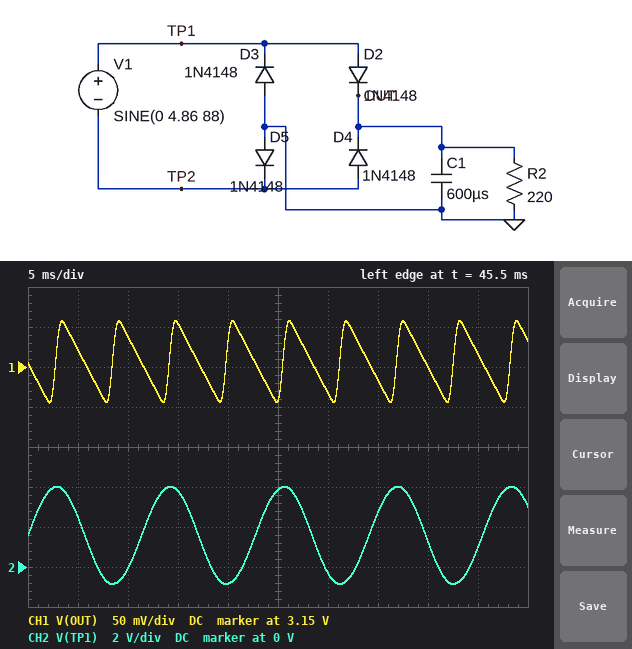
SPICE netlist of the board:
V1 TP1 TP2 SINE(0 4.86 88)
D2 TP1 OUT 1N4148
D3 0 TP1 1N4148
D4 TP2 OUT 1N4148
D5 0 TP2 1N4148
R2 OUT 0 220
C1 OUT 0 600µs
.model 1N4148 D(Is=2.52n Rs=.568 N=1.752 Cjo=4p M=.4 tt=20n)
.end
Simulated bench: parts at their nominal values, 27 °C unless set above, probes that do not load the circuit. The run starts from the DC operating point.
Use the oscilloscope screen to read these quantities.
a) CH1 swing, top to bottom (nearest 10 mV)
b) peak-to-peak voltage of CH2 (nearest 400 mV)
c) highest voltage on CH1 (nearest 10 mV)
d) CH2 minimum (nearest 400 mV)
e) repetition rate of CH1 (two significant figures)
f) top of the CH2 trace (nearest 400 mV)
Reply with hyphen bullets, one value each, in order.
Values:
- 100 mV
- 4.8 V
- 3.21 V
- -800 mV
- 180 Hz
- 4.0 V
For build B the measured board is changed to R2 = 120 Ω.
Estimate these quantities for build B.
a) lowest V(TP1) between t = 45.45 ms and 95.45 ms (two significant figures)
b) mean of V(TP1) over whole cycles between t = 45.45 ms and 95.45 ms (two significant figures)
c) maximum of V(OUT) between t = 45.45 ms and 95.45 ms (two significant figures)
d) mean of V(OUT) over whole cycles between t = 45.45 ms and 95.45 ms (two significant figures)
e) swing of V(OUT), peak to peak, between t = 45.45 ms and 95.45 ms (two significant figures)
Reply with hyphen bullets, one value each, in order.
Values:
- -900 mV
- 1.5 V
- 3.1 V
- 3.0 V
- 180 mV
